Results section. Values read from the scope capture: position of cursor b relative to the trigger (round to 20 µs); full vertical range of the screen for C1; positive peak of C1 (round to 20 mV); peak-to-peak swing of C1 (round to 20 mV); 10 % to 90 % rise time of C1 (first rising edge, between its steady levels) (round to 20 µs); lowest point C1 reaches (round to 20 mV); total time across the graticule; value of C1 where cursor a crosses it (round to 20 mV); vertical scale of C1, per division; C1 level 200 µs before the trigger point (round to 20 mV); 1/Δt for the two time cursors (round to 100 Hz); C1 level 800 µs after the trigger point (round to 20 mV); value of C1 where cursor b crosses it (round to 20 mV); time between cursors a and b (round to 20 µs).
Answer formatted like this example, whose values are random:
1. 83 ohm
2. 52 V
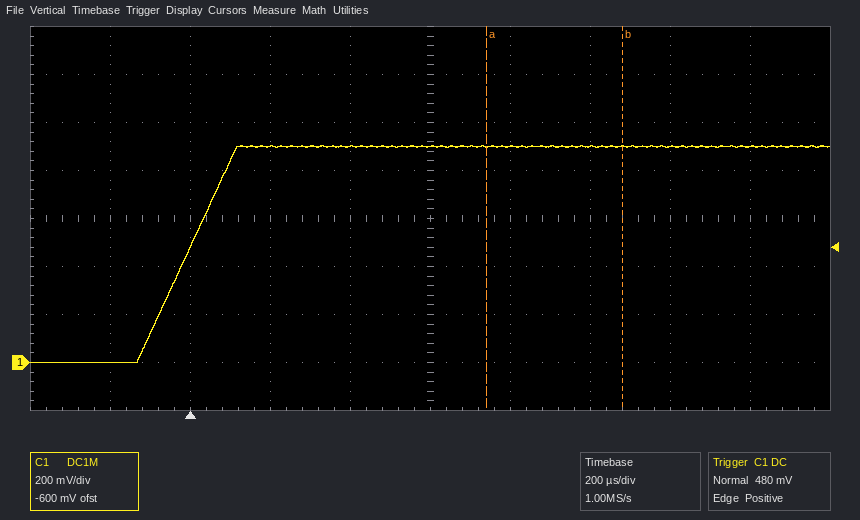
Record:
1. +1.08 ms
2. 1.6 V
3. 900 mV
4. 900 mV
5. 200 µs
6. 0 mV
7. 2 ms
8. 900 mV
9. 200 mV
10. 0 mV
11. 2.9 kHz
12. 900 mV
13. 900 mV
14. 340 µs
